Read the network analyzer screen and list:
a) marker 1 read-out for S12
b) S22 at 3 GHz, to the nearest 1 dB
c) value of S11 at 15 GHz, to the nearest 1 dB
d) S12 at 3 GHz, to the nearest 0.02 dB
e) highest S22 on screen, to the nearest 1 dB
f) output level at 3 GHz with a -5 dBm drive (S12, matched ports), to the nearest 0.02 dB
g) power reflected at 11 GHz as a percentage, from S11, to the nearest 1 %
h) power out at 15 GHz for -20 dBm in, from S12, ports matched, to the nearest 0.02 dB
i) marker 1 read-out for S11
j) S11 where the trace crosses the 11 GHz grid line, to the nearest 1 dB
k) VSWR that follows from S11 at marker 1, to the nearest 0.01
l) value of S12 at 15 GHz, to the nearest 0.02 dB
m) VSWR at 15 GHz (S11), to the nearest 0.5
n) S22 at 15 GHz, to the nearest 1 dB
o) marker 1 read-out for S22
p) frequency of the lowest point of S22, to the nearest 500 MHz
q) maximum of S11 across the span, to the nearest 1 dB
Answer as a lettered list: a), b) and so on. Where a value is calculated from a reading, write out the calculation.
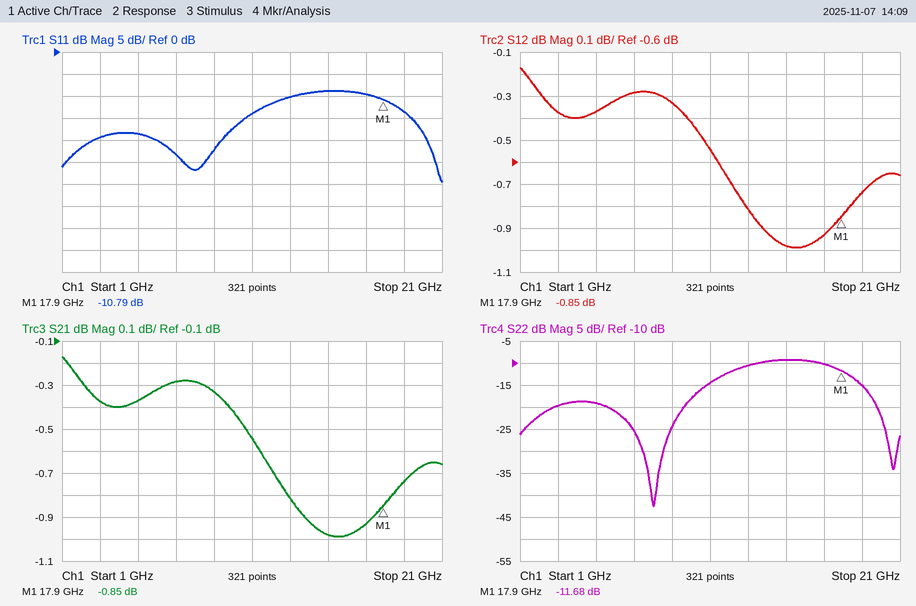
a) -0.85 dB
b) -20 dB
c) -9 dB
d) -0.38 dB
e) -9 dB
f) -5 dBm + (-0.38 dB) = -5.38 dBm
g) 10^(-14/10) ≈ 4 %
h) -20 dBm + (-0.98 dB) = -20.98 dBm
i) -10.79 dB
j) -14 dB
k) (1 + 0.2887)/(1 − 0.2887) ≈ 1.81
l) -0.98 dB
m) |Γ| = 10^(-9/20) = 0.3548; VSWR = (1 + 0.3548)/(1 − 0.3548) ≈ 2.10, so 2.0 to the nearest 0.5
n) -9 dB
o) -11.68 dB
p) 8.0 GHz
q) -9 dB
